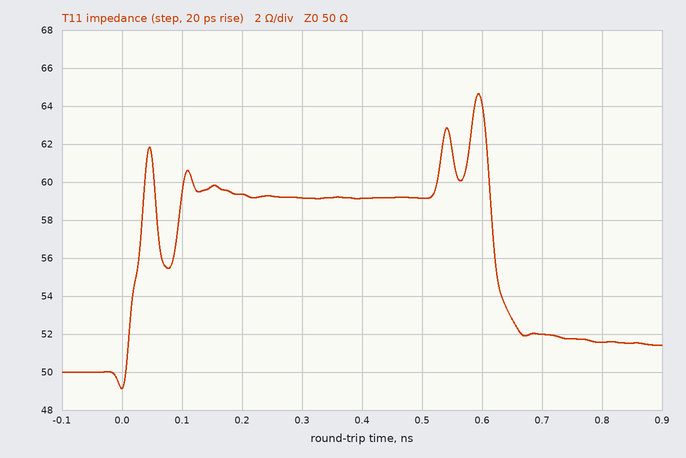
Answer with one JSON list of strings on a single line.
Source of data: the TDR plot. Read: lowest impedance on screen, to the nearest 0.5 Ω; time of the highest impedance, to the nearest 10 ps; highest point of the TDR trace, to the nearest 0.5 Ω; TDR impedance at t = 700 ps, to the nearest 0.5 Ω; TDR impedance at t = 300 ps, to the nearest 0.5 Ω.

["49.0 Ω", "590 ps", "64.5 Ω", "52.0 Ω", "59.0 Ω"]
